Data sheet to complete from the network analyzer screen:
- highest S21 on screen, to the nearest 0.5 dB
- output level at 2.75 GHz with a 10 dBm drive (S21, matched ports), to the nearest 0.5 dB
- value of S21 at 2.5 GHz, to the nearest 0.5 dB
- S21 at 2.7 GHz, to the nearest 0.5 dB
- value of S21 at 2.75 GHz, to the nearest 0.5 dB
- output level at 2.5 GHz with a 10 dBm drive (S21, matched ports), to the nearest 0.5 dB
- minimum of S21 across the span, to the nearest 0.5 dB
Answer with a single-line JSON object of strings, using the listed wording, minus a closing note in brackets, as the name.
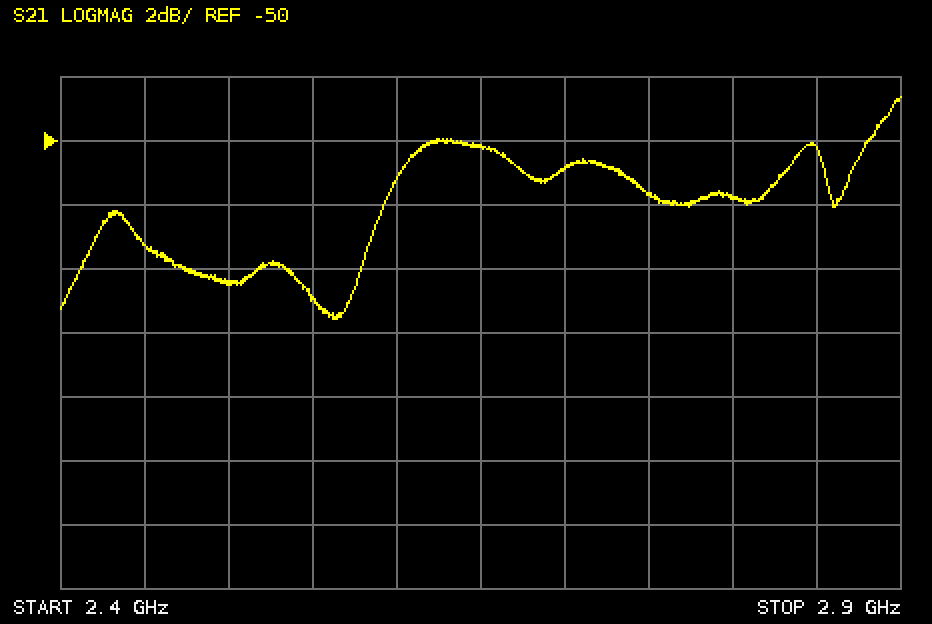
{"highest S21 on screen, to the nearest 0.5 dB": "-48.5 dB", "output level at 2.75 GHz with a 10 dBm drive (S21, matched ports), to the nearest 0.5 dB": "-41.5 dBm", "value of S21 at 2.5 GHz, to the nearest 0.5 dB": "-54.5 dB", "S21 at 2.7 GHz, to the nearest 0.5 dB": "-51.0 dB", "value of S21 at 2.75 GHz, to the nearest 0.5 dB": "-51.5 dB", "output level at 2.5 GHz with a 10 dBm drive (S21, matched ports), to the nearest 0.5 dB": "-44.5 dBm", "minimum of S21 across the span, to the nearest 0.5 dB": "-55.5 dB"}
